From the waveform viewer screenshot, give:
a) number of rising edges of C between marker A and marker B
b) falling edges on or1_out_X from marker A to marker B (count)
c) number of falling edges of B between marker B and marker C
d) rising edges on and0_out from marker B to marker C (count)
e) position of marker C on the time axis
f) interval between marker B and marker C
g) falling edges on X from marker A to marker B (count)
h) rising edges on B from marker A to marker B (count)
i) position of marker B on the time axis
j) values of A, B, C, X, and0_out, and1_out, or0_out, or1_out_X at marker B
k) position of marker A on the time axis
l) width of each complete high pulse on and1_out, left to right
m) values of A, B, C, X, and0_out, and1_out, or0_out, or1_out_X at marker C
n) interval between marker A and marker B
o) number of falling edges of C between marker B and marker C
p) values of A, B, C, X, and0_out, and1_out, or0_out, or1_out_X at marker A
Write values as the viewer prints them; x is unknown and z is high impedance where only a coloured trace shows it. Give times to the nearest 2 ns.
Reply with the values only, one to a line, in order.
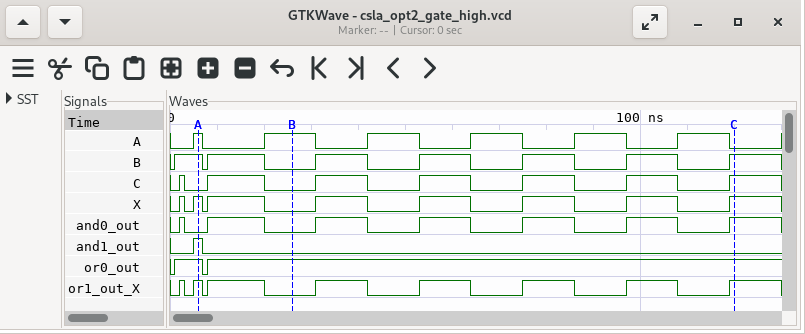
1
2
4
5
120 ns
94 ns
2
1
26 ns
A=1, B=0, C=0, X=0, and0_out=0, and1_out=0, or0_out=1, or1_out_X=0
6 ns
2 ns
A=0, B=1, C=1, X=1, and0_out=1, and1_out=0, or0_out=1, or1_out_X=1
20 ns
4
A=1, B=1, C=0, X=1, and0_out=0, and1_out=1, or0_out=1, or1_out_X=1
